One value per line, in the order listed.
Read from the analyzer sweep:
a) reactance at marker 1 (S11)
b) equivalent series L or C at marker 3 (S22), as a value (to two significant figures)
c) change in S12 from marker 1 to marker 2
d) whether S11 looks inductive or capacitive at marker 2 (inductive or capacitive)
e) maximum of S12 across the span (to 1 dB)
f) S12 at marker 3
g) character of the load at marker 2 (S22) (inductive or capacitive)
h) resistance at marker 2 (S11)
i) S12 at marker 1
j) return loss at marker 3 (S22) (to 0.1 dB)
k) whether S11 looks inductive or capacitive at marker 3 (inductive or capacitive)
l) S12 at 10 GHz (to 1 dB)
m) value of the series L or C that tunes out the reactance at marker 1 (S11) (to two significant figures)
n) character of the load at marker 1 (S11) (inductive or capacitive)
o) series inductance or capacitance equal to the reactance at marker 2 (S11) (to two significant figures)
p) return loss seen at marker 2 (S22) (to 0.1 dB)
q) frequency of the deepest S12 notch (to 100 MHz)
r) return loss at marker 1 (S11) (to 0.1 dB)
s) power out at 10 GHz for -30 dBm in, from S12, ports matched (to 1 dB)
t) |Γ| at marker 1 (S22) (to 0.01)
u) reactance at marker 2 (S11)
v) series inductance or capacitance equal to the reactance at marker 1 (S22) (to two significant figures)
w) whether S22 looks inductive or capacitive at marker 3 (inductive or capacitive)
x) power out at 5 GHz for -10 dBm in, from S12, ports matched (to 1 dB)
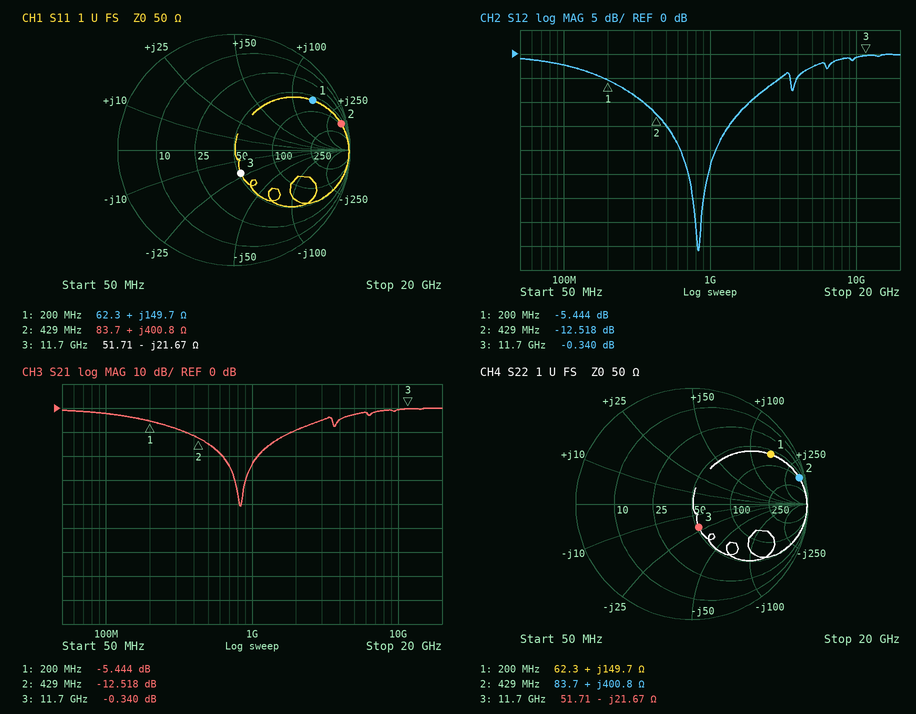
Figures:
+149.7 Ω
630 fF
-7.074 dB
inductive
0 dB
-0.340 dB
inductive
83.7 Ω
-5.444 dB
13.6 dB
capacitive
-1 dB
5.3 pF
inductive
150 nH
0.4 dB
800 MHz
1.9 dB
-31 dBm
0.80
+400.8 Ω
120 nH
capacitive
-13 dBm
